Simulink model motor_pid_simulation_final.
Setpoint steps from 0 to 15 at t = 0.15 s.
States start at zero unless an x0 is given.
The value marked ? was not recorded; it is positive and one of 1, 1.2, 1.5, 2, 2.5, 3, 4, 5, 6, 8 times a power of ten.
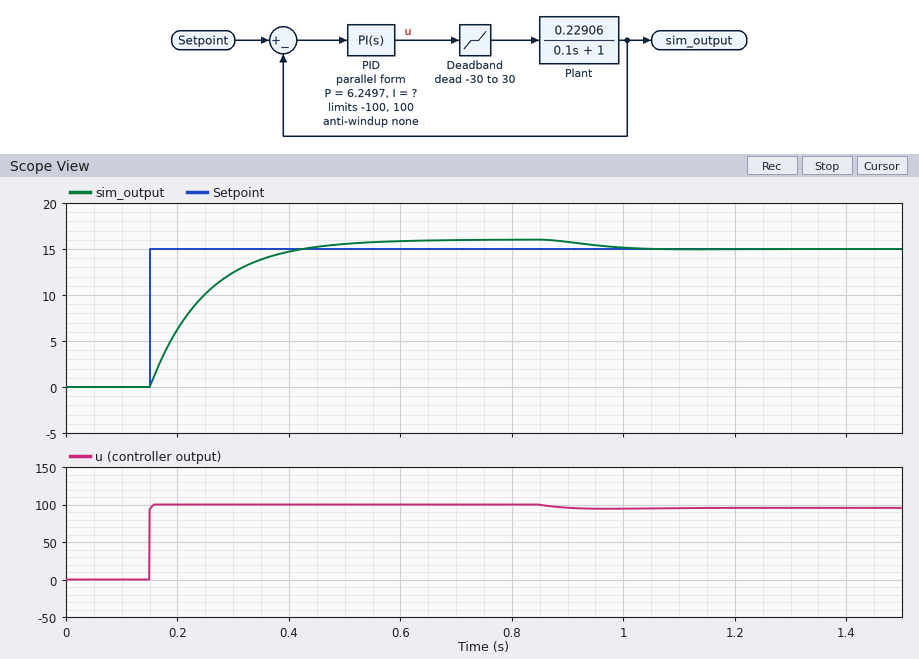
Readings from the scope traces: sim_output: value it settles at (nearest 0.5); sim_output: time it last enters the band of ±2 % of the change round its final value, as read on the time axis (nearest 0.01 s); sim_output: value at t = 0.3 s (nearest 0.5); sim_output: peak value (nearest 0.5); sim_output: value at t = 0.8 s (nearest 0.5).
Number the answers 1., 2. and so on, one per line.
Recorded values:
1. 15.0
2. 0.97 s
3. 12.5
4. 16.0
5. 16.0
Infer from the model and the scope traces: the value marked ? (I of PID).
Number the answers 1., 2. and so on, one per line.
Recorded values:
1. 120
